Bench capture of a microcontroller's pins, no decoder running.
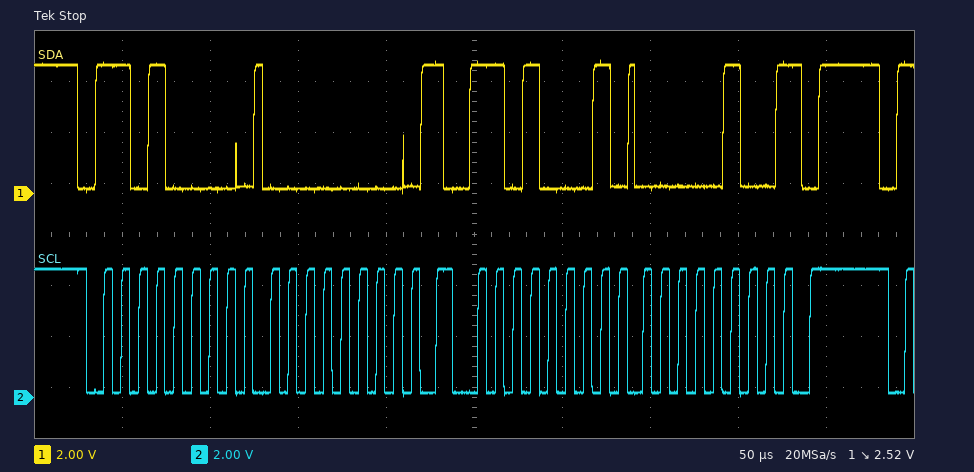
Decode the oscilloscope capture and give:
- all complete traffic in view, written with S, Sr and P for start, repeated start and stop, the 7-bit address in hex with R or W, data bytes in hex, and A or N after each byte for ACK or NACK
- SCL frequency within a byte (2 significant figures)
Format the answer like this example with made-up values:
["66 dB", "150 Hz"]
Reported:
["S 68W A 00 A Sr 68R A 04 N P", "100 kHz"]
